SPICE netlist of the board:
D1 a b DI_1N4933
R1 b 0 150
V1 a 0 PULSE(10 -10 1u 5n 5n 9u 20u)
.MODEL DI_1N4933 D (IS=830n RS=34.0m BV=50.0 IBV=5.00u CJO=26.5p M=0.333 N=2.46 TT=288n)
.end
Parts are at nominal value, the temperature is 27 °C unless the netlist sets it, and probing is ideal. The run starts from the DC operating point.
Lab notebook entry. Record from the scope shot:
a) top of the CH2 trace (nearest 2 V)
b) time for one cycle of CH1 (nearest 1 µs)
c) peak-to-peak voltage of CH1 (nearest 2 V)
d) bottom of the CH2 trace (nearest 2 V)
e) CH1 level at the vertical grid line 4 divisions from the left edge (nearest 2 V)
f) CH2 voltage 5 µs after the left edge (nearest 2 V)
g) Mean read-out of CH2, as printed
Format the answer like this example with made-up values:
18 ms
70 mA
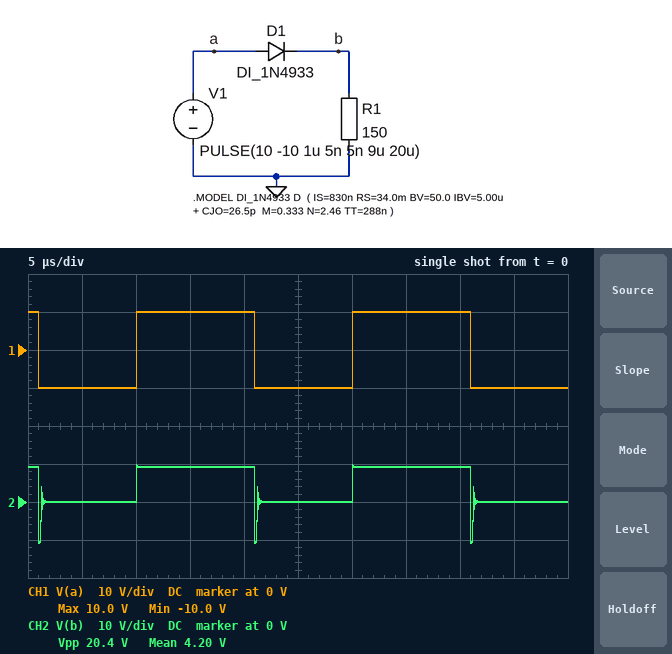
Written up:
10 V
20 µs
20 V
-10 V
10 V
0 V
4.20 V
